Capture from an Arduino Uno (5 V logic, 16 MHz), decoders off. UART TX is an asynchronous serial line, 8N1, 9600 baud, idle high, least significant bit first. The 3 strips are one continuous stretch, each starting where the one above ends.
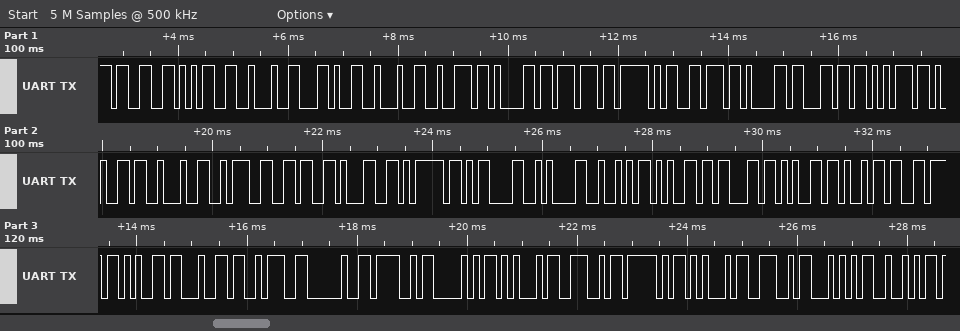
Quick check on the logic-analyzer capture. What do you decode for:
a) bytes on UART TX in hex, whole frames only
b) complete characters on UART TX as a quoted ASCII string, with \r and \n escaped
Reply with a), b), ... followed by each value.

a) 0x33 0x35 0x22 0x2C 0x22 0x72 0x61 0x77 0x5F 0x76 0x61 0x6C 0x75 0x65 0x22 0x3A 0x36 0x31 0x7D 0x0D 0x0A 0x52 0x65 0x63 0x65 0x69 0x76 0x65 0x64 0x3A 0x20 0x4F 0x50 0x45 0x4E 0x5F 0x45 0x4E 0x54 0x52
b) "35\",\"raw_value\":61}\r\nReceived: OPEN_ENTR"
